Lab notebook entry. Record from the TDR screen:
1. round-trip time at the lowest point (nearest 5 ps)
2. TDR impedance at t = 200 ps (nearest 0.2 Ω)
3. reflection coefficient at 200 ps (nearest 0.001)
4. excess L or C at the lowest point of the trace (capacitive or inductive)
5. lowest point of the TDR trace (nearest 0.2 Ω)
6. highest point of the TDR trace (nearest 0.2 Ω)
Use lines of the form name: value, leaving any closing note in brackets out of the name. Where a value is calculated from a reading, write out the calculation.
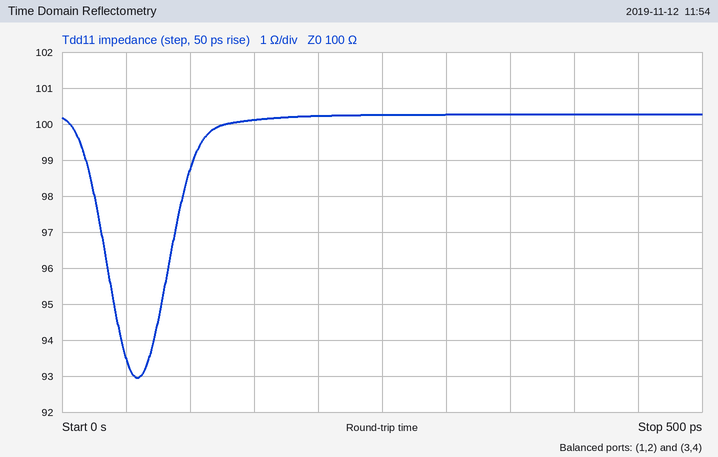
round-trip time at the lowest point: 60 ps
TDR impedance at t = 200 ps: 100.2 Ω
reflection coefficient at 200 ps: (100.2 − 100)/(100.2 + 100) ≈ +0.001
excess L or C at the lowest point of the trace: capacitive
lowest point of the TDR trace: 93.0 Ω
highest point of the TDR trace: 100.2 Ω
